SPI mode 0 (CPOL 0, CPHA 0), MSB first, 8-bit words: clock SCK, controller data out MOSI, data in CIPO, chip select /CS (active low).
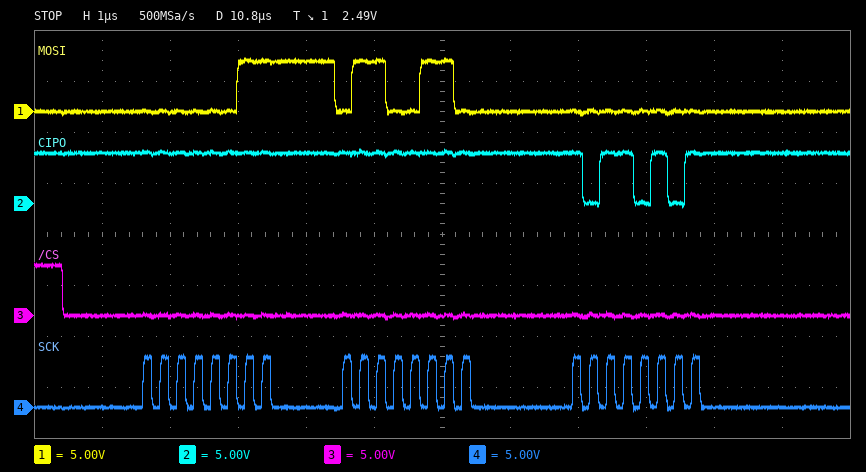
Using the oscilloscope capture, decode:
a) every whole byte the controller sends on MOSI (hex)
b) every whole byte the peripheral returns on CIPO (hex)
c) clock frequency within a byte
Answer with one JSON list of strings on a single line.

["0x03 0x66 0x00", "0xFF 0xFF 0xB5", "4 MHz"]
